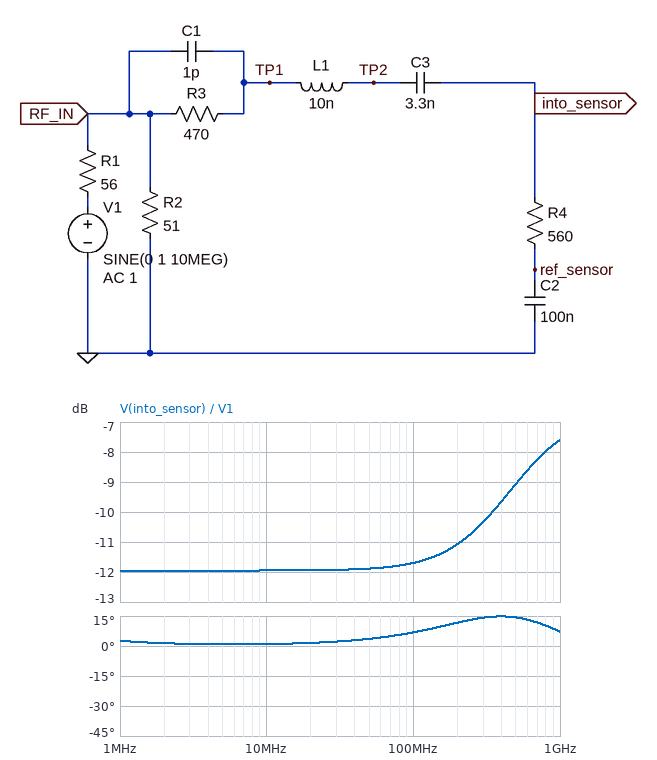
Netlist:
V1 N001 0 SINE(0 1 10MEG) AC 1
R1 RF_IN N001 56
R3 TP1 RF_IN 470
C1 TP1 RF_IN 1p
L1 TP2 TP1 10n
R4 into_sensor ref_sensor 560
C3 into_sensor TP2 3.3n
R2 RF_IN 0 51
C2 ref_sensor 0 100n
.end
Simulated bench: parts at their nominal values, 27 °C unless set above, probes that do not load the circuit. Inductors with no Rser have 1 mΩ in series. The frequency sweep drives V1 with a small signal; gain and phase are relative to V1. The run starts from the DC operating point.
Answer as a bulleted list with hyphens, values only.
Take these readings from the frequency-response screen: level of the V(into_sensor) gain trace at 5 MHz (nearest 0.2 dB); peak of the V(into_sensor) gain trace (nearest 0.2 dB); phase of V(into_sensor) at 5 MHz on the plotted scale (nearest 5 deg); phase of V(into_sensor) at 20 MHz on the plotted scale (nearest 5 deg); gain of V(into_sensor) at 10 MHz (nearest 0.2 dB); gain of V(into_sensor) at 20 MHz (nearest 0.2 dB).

- -12.0 dB
- -7.6 dB
- 0 deg
- 0 deg
- -12.0 dB
- -12.0 dB
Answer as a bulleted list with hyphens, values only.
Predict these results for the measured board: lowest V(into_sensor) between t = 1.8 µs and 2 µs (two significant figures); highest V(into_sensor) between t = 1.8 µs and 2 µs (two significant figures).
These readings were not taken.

- -250 mV
- 250 mV
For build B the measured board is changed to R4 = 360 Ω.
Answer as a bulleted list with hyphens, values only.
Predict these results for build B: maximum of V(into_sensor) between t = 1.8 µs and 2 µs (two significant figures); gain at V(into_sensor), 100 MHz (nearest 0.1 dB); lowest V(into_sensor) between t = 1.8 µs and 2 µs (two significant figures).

- 200 mV
- -13.7 dB
- -200 mV
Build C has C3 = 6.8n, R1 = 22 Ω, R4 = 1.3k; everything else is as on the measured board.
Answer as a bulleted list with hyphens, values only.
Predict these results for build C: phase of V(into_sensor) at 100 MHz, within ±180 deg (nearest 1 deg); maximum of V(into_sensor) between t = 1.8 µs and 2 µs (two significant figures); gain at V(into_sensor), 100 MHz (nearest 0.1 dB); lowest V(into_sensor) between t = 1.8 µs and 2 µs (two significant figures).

- 4 deg
- 510 mV
- -5.7 dB
- -510 mV
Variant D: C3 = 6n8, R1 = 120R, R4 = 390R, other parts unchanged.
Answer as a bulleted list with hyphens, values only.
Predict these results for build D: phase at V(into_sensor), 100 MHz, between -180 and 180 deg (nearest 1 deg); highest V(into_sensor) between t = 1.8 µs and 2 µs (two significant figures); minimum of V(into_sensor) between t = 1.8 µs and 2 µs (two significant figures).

- 8 deg
- 130 mV
- -130 mV
